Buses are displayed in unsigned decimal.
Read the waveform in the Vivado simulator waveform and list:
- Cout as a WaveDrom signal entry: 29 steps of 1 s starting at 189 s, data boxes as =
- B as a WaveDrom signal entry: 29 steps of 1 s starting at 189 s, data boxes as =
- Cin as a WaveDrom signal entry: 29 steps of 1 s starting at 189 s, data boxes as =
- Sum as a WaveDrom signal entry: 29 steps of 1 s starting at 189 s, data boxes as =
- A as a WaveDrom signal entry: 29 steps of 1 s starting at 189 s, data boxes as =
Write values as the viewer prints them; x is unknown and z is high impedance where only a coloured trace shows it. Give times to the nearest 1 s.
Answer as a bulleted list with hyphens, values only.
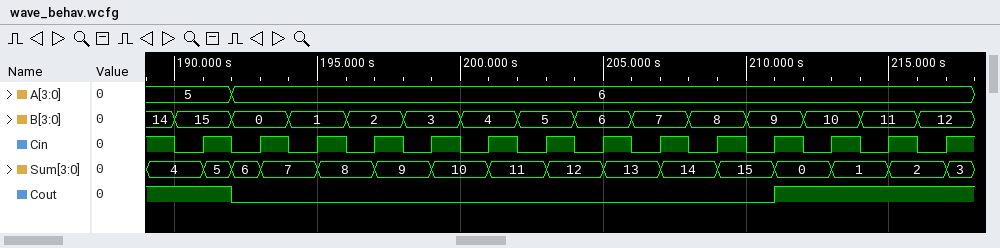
- {name: 'Cout', wave: '1..0..................1......'}
- {name: 'B', wave: '==.=.=.=.=.=.=.=.=.=.=.=.=.=.', data: '14 15 0 1 2 3 4 5 6 7 8 9 10 11 12'}
- {name: 'Cin', wave: '10101010101010101010101010101'}
- {name: 'Sum', wave: '=.===.=.=.=.=.=.=.=.=.=.=.=.=', data: '4 5 6 7 8 9 10 11 12 13 14 15 0 1 2 3'}
- {name: 'A', wave: '=..=.........................', data: '5 6'}
